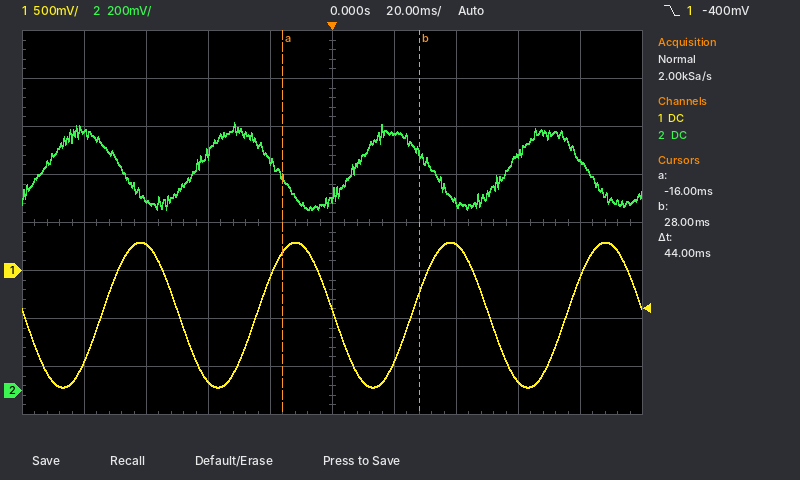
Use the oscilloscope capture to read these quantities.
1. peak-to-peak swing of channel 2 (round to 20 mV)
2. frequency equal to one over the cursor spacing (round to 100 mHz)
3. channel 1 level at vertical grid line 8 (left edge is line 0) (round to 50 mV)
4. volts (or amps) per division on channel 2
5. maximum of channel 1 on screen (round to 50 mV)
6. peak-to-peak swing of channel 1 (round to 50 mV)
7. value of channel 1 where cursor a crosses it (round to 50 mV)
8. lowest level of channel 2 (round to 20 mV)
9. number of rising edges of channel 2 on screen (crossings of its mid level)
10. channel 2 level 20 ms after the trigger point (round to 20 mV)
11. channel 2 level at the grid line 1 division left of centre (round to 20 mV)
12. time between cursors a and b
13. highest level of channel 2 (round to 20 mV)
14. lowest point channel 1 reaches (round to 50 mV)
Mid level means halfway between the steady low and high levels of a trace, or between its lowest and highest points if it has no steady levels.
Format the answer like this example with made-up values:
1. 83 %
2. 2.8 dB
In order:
1. 360 mV
2. 22.7 Hz
3. -1.15 V
4. 200 mV
5. 300 mV
6. 1.50 V
7. 200 mV
8. 760 mV
9. 4
10. 1.08 V
11. 960 mV
12. 44 ms
13. 1.12 V
14. -1.20 V
